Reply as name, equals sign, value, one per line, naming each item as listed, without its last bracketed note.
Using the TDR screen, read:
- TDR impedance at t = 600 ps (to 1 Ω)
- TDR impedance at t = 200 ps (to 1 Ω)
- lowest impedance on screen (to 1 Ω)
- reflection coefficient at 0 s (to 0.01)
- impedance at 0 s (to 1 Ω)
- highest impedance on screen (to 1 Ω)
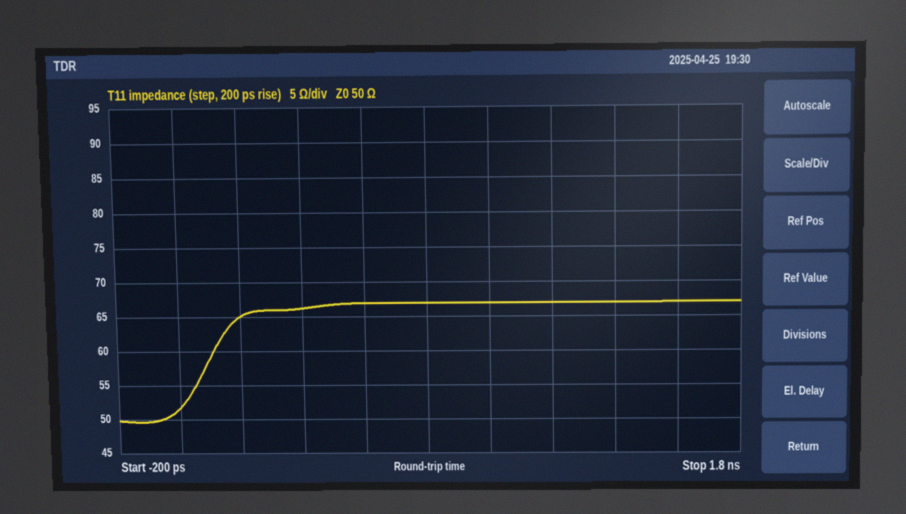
TDR impedance at t = 600 ps = 67 Ω
TDR impedance at t = 200 ps = 65 Ω
lowest impedance on screen = 50 Ω
reflection coefficient at 0 s = +0.02
impedance at 0 s = 52 Ω
highest impedance on screen = 67 Ω
